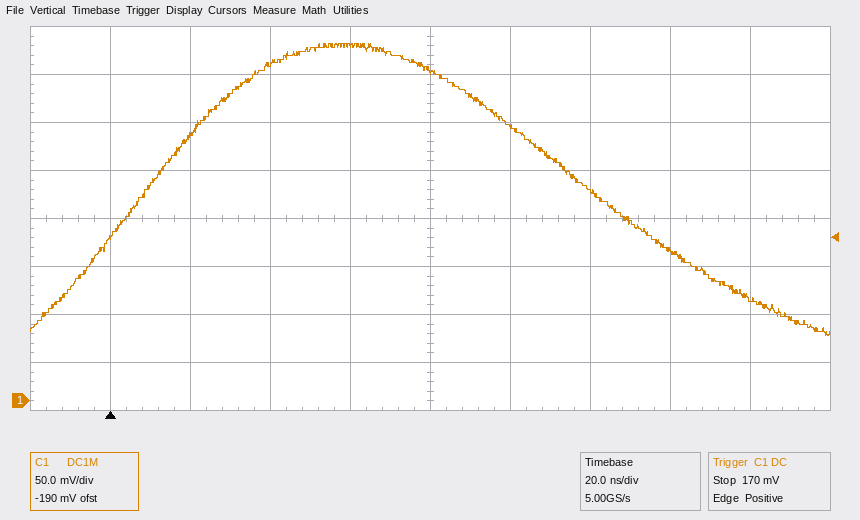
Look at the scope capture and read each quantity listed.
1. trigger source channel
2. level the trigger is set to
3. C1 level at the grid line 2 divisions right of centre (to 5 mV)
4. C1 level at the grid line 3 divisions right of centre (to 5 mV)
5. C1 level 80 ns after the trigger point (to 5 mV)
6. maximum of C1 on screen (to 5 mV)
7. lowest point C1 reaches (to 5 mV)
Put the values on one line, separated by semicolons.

C1; 170 mV; 220 mV; 155 mV; 345 mV; 370 mV; 70 mV
